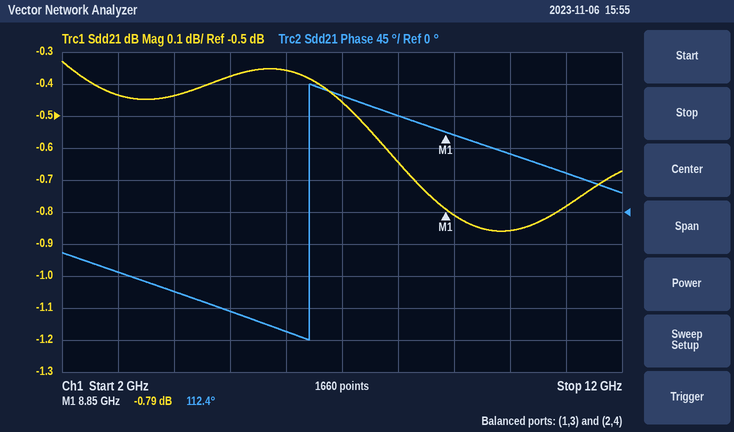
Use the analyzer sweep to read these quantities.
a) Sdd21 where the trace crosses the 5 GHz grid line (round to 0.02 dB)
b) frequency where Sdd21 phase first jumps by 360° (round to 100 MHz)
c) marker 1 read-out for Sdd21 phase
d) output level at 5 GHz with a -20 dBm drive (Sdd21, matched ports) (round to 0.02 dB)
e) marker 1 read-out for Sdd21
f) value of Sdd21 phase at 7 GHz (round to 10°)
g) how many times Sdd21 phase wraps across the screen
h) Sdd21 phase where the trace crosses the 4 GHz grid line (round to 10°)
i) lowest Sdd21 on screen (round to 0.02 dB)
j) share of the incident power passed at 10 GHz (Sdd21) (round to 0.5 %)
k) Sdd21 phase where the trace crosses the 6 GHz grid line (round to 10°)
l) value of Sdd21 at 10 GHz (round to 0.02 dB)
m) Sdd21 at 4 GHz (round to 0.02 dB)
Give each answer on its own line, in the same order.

-0.38 dB
6.4 GHz
112.4°
-20.38 dBm
-0.79 dB
160°
1
-110°
-0.86 dB
82.0 %
-170°
-0.86 dB
-0.44 dB
